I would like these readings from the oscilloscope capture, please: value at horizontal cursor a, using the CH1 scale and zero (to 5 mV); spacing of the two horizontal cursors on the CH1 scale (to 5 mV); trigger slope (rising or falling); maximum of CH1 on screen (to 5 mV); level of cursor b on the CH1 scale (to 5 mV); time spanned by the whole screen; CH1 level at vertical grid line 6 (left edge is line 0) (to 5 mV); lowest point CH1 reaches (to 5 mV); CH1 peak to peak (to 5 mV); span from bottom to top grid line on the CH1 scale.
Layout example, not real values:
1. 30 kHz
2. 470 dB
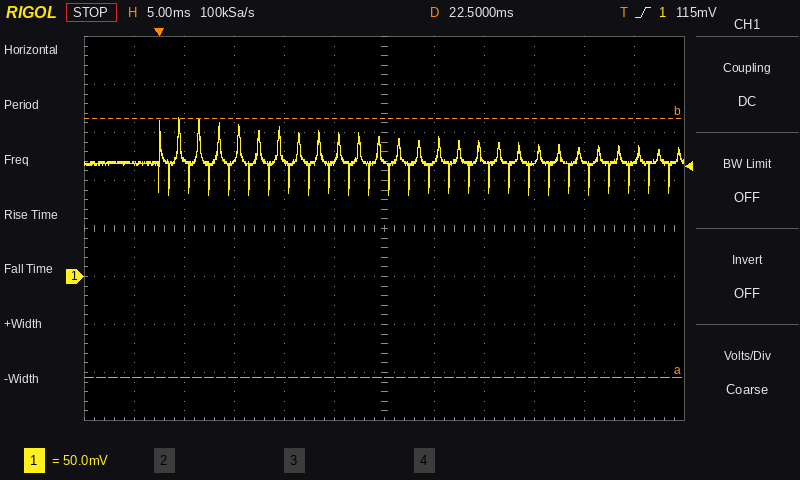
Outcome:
1. -105 mV
2. 270 mV
3. rising
4. 165 mV
5. 165 mV
6. 60 ms
7. 120 mV
8. 85 mV
9. 80 mV
10. 400 mV
